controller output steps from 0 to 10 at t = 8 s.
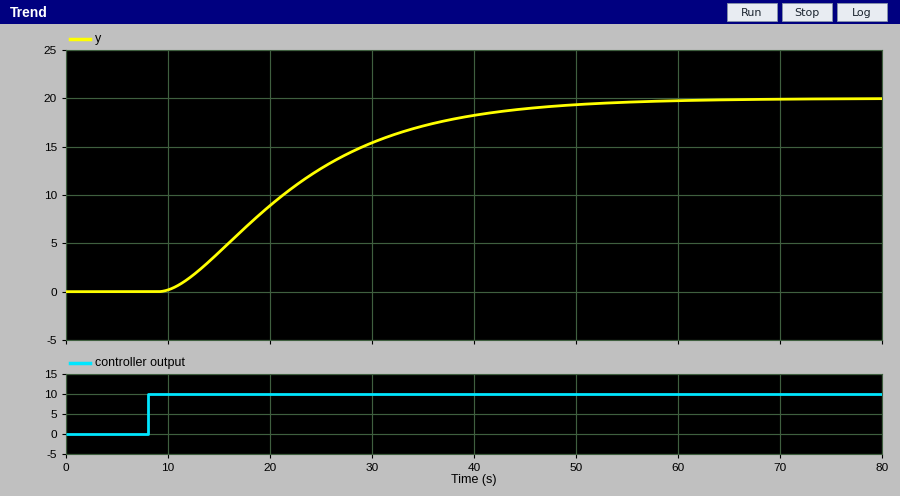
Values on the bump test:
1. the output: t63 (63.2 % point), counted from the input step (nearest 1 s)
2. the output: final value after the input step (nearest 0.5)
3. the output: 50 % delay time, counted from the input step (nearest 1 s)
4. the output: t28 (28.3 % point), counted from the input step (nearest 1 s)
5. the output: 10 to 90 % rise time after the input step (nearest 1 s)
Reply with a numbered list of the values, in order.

1. 17 s
2. 20.0
3. 13 s
4. 9 s
5. 26 s
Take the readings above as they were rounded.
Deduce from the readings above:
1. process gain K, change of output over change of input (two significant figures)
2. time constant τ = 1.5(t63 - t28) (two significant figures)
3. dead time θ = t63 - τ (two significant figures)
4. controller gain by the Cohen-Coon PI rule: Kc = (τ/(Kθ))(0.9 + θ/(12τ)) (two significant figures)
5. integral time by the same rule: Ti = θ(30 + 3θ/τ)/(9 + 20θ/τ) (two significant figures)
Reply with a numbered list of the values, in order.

1. 2.0
2. 12 s
3. 5.0 s
4. 1.1
5. 9.0 s
